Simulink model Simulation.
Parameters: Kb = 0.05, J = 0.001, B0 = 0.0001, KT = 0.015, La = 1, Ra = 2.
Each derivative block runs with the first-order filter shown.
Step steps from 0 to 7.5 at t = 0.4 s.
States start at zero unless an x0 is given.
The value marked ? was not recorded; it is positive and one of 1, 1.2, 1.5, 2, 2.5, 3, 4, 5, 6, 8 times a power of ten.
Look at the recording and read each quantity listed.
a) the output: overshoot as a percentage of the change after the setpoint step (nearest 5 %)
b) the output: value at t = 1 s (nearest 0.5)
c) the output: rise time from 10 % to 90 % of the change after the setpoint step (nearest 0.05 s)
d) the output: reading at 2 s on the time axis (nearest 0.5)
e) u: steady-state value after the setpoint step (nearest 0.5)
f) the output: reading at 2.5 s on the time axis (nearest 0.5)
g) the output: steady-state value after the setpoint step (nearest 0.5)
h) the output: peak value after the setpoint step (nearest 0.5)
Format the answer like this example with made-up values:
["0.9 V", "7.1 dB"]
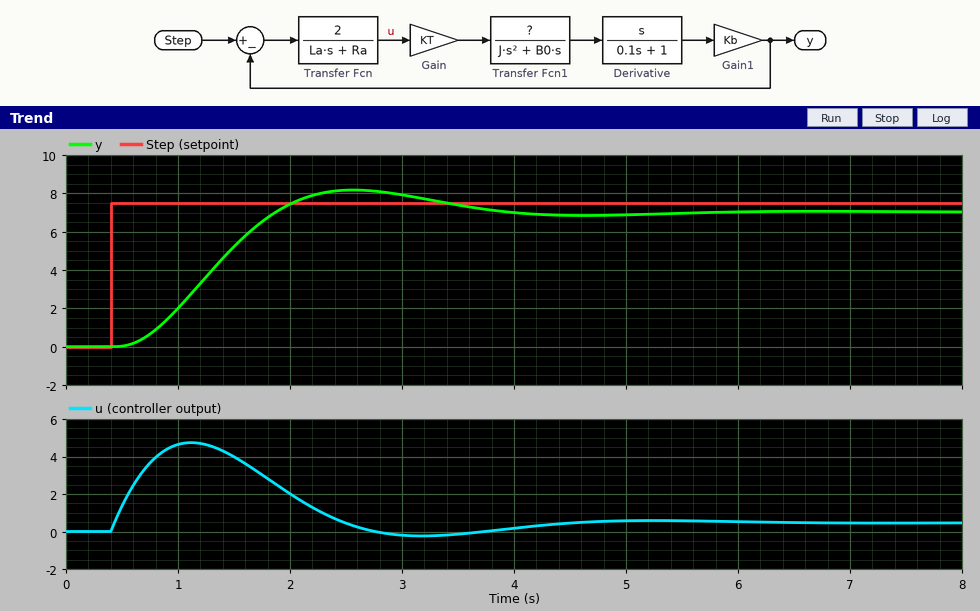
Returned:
["15 %", "2.0", "0.95 s", "7.5", "0.5", "8.0", "7.0", "8.0"]
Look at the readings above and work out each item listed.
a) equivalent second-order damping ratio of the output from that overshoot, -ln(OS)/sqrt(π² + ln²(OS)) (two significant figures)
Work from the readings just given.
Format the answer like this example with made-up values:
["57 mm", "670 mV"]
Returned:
["0.52"]
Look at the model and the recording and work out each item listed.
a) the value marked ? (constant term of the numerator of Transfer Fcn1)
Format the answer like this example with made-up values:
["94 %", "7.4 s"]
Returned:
["2"]
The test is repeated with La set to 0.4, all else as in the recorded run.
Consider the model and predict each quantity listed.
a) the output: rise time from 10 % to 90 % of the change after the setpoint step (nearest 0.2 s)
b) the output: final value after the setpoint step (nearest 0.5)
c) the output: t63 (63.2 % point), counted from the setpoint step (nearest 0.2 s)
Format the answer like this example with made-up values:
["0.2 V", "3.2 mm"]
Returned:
["0.8 s", "7.0", "0.8 s"]
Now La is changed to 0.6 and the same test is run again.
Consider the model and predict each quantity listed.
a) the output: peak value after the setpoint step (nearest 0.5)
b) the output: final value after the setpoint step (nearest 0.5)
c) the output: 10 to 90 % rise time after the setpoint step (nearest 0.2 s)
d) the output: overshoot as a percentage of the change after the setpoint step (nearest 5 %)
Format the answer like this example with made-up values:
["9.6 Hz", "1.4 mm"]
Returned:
["7.5", "7.0", "0.8 s", "10 %"]
